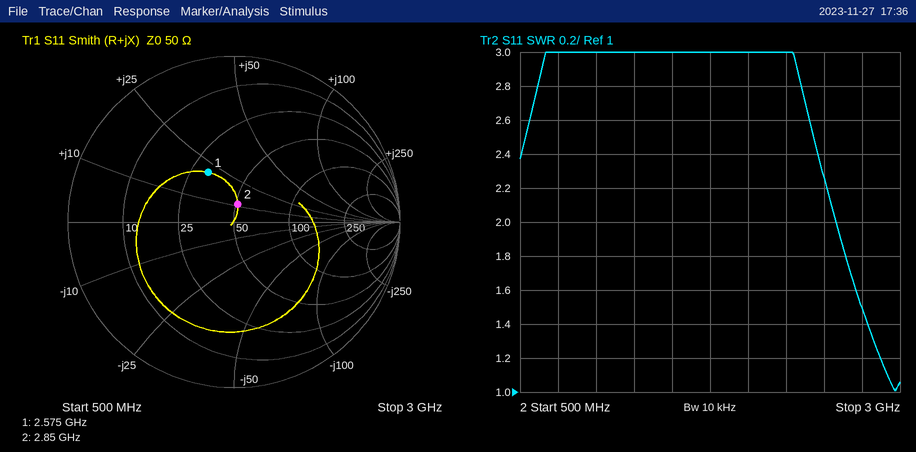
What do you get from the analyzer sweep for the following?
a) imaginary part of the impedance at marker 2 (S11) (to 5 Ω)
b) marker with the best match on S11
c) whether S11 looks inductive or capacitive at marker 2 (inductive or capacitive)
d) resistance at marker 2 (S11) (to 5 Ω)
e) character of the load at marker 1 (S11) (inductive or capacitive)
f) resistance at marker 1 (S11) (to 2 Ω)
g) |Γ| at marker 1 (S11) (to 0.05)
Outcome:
+10 Ω
marker 2
inductive
50 Ω
inductive
32 Ω
0.35
